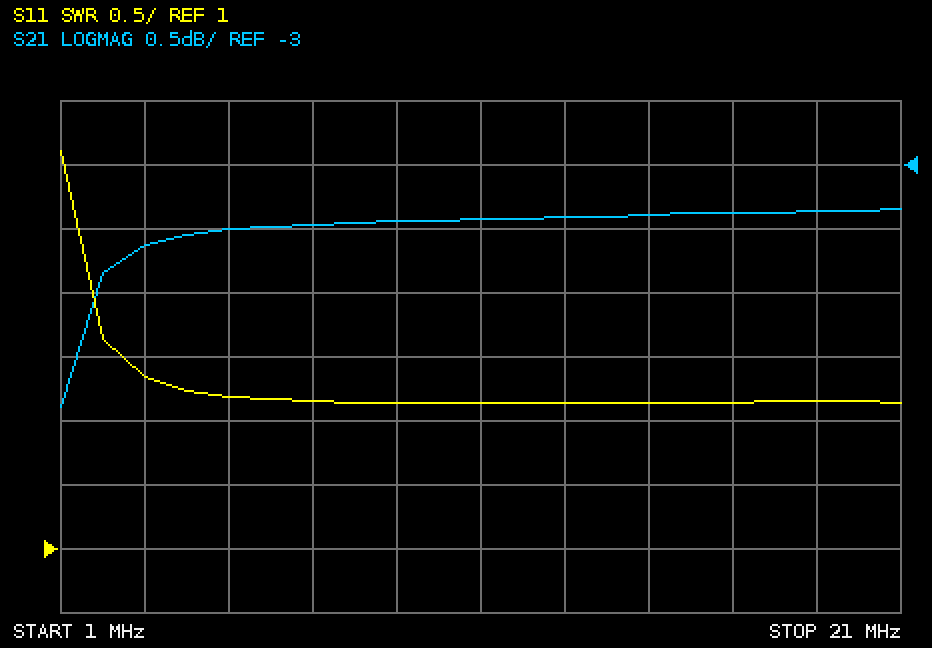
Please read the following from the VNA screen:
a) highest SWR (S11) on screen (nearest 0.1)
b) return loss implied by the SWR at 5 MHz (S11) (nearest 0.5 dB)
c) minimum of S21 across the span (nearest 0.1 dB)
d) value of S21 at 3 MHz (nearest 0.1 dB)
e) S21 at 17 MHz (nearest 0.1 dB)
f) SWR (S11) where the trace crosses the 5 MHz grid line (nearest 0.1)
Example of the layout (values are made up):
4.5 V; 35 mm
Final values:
4.1; 8.5 dB; -4.9 dB; -3.6 dB; -3.4 dB; 2.2
